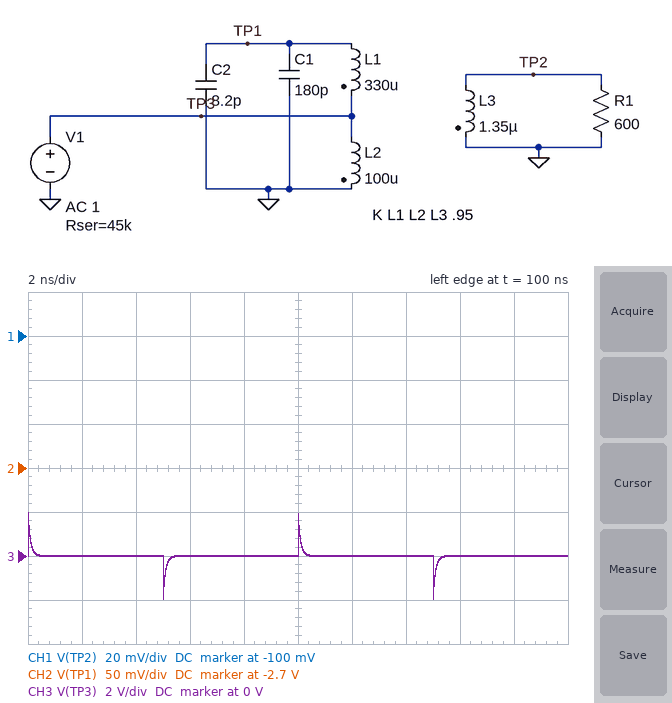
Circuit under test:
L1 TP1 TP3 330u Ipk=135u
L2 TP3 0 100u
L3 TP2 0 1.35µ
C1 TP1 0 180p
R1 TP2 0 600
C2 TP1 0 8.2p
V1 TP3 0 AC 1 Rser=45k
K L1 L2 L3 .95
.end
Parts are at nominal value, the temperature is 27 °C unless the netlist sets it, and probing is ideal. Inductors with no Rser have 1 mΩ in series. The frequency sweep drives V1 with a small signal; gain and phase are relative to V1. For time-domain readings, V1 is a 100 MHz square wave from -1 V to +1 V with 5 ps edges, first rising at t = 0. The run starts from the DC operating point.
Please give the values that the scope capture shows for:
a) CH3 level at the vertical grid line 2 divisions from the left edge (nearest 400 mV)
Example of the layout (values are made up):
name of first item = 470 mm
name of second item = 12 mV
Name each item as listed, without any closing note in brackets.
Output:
CH3 level at the vertical grid line 2 divisions from the left edge = 0 V
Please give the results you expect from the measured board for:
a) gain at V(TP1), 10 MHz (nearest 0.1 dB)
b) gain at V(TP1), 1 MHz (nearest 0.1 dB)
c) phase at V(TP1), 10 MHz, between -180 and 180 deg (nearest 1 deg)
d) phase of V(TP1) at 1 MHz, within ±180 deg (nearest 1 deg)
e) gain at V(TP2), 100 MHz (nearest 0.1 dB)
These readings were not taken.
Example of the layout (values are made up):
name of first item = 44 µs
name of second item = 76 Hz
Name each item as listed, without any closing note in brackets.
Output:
gain at V(TP1), 10 MHz = -63.6 dB
gain at V(TP1), 1 MHz = -41.9 dB
phase at V(TP1), 10 MHz, between -180 and 180 deg = -90 deg
phase of V(TP1) at 1 MHz, within ±180 deg = -90 deg
gain at V(TP2), 100 MHz = -56.7 dB
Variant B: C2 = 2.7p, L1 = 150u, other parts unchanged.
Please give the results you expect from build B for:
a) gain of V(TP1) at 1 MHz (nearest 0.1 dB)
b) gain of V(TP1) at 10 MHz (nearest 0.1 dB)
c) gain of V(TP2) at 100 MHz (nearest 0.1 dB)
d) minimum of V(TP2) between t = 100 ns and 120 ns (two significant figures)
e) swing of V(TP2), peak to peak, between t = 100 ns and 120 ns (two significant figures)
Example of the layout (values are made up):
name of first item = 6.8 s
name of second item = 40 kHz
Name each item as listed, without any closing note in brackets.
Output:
gain of V(TP1) at 1 MHz = -38.3 dB
gain of V(TP1) at 10 MHz = -61.2 dB
gain of V(TP2) at 100 MHz = -67.3 dB
minimum of V(TP2) between t = 100 ns and 120 ns = -4.2 mV
swing of V(TP2), peak to peak, between t = 100 ns and 120 ns = 9.1 mV
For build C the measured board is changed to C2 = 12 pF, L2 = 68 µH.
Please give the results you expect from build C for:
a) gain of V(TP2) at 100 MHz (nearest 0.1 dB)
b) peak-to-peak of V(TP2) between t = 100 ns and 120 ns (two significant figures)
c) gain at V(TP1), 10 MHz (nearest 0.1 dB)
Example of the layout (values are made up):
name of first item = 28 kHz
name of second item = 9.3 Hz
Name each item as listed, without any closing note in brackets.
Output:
gain of V(TP2) at 100 MHz = -55.6 dB
peak-to-peak of V(TP2) between t = 100 ns and 120 ns = 33 mV
gain at V(TP1), 10 MHz = -64.9 dB
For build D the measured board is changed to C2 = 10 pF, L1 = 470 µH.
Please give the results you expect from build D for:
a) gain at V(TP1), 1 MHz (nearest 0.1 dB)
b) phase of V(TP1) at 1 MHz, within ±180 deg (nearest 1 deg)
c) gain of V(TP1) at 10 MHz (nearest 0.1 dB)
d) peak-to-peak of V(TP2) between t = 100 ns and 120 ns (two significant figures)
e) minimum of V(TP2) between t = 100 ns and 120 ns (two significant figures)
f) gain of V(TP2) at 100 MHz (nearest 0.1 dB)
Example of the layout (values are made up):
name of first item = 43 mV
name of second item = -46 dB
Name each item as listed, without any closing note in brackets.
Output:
gain at V(TP1), 1 MHz = -43.5 dB
phase of V(TP1) at 1 MHz, within ±180 deg = -90 deg
gain of V(TP1) at 10 MHz = -64.7 dB
peak-to-peak of V(TP2) between t = 100 ns and 120 ns = 34 mV
minimum of V(TP2) between t = 100 ns and 120 ns = -17 mV
gain of V(TP2) at 100 MHz = -54.1 dB
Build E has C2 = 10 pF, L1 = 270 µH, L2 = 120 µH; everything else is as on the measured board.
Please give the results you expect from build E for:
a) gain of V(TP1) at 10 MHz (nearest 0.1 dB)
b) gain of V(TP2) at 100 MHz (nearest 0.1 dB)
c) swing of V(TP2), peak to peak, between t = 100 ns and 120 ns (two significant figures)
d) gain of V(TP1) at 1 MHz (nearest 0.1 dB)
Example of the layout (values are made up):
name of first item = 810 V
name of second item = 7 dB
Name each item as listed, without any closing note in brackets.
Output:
gain of V(TP1) at 10 MHz = -62.6 dB
gain of V(TP2) at 100 MHz = -59.8 dB
swing of V(TP2), peak to peak, between t = 100 ns and 120 ns = 19 mV
gain of V(TP1) at 1 MHz = -40.9 dB
